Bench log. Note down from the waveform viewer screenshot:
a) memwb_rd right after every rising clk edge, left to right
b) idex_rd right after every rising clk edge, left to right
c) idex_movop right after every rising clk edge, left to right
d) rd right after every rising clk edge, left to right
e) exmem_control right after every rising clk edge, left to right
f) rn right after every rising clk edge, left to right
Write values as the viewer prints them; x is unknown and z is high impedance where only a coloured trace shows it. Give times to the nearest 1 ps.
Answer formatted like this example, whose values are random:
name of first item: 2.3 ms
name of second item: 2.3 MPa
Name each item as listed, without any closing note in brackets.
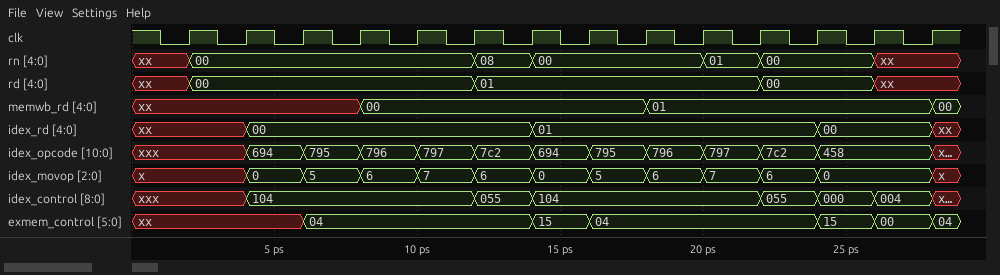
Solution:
memwb_rd right after every rising clk edge, left to right: xx, xx, xx, 00, 00, 00, 00, 00, 01, 01, 01, 01, 01, 00
idex_rd right after every rising clk edge, left to right: xx, 00, 00, 00, 00, 00, 01, 01, 01, 01, 01, 00, 00, xx
idex_movop right after every rising clk edge, left to right: x, 0, 5, 6, 7, 6, 0, 5, 6, 7, 6, 0, 0, x
rd right after every rising clk edge, left to right: 00, 00, 00, 00, 00, 01, 01, 01, 01, 01, 00, 00, xx, xx
exmem_control right after every rising clk edge, left to right: xx, xx, 04, 04, 04, 04, 15, 04, 04, 04, 04, 15, 00, 04
rn right after every rising clk edge, left to right: 00, 00, 00, 00, 00, 08, 00, 00, 00, 01, 00, 00, xx, xx
